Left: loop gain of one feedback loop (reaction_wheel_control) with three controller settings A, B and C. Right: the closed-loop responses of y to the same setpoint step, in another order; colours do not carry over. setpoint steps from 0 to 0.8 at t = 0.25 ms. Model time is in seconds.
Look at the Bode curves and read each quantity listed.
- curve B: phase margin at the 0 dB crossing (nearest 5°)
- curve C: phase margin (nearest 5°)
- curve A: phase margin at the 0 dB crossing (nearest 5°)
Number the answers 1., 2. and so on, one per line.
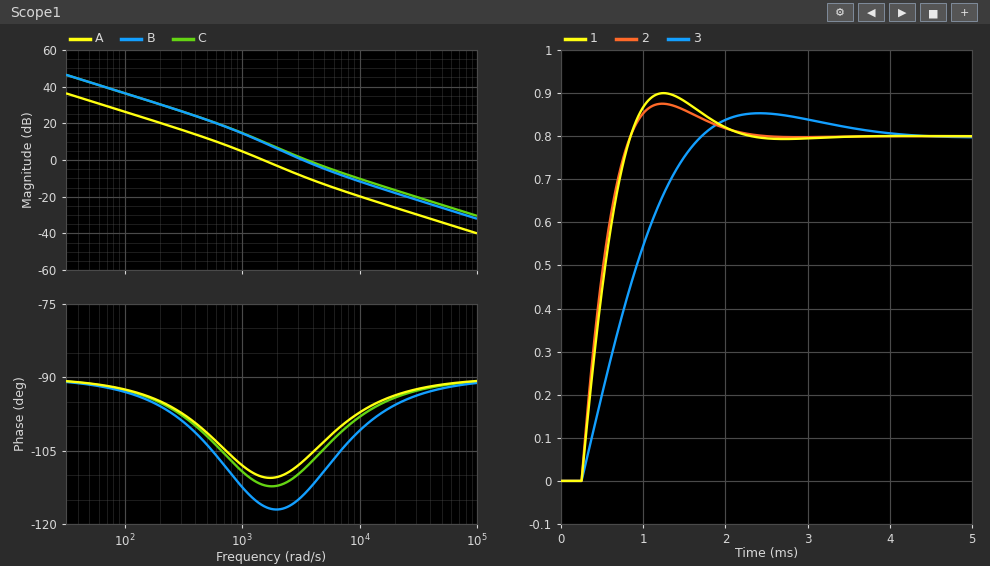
1. 65°
2. 70°
3. 70°
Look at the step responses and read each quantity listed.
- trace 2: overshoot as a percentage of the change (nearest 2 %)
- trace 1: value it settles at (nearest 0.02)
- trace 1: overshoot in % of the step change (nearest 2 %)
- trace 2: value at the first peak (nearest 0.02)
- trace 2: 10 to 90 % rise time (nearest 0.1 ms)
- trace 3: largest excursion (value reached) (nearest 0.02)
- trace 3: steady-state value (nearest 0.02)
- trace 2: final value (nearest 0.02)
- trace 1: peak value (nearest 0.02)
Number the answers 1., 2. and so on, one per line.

1. 10 %
2. 0.80
3. 12 %
4. 0.88
5. 0.4 ms
6. 0.86
7. 0.80
8. 0.80
9. 0.90
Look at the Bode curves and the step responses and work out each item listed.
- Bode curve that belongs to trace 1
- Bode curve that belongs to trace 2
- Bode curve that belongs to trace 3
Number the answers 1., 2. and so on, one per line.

1. B
2. C
3. A
